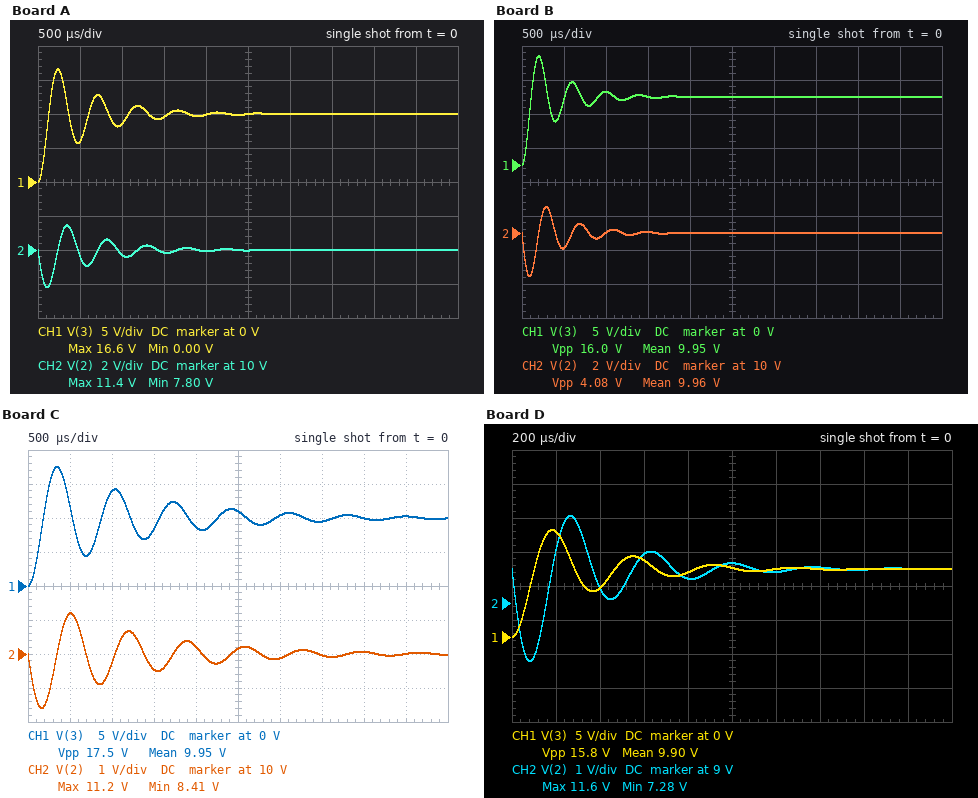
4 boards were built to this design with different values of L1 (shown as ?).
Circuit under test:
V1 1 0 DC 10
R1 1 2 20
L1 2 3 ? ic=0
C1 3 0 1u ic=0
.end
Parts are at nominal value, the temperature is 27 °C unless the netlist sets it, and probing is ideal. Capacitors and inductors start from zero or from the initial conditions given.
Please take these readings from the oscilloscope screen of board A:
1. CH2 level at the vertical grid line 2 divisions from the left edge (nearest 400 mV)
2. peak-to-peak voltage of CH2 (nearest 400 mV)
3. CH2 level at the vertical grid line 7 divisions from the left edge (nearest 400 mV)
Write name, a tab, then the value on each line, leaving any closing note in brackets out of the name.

CH2 level at the vertical grid line 2 divisions from the left edge	9.6 V
peak-to-peak voltage of CH2	3.6 V
CH2 level at the vertical grid line 7 divisions from the left edge	10.0 V
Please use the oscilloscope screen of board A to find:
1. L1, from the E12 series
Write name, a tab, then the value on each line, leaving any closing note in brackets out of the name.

L1, from the E12 series	5.6 mH
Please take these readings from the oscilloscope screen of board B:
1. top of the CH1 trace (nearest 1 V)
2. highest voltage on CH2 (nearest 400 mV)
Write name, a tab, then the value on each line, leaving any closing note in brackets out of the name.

top of the CH1 trace	16 V
highest voltage on CH2	11.6 V
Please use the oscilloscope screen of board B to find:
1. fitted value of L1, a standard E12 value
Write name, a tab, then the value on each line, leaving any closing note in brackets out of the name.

fitted value of L1, a standard E12 value	3.9 mH
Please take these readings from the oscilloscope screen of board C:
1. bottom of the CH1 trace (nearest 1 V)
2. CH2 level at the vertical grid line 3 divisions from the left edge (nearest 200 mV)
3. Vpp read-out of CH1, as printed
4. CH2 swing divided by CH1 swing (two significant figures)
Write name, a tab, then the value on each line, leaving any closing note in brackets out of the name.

bottom of the CH1 trace	0 V
CH2 level at the vertical grid line 3 divisions from the left edge	9.6 V
Vpp read-out of CH1, as printed	17.5 V
CH2 swing divided by CH1 swing	0.16
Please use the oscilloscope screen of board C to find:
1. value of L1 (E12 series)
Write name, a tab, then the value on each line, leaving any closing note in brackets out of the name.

value of L1	12 mH
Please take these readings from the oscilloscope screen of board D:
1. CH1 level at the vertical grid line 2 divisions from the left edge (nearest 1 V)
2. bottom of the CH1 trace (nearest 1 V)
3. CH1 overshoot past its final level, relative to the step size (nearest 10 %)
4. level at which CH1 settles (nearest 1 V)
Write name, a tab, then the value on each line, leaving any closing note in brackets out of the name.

CH1 level at the vertical grid line 2 divisions from the left edge	7 V
bottom of the CH1 trace	0 V
CH1 overshoot past its final level, relative to the step size	60 %
level at which CH1 settles	10 V
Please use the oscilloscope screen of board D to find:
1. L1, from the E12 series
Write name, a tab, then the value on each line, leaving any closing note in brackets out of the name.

L1, from the E12 series	3.3 mH
